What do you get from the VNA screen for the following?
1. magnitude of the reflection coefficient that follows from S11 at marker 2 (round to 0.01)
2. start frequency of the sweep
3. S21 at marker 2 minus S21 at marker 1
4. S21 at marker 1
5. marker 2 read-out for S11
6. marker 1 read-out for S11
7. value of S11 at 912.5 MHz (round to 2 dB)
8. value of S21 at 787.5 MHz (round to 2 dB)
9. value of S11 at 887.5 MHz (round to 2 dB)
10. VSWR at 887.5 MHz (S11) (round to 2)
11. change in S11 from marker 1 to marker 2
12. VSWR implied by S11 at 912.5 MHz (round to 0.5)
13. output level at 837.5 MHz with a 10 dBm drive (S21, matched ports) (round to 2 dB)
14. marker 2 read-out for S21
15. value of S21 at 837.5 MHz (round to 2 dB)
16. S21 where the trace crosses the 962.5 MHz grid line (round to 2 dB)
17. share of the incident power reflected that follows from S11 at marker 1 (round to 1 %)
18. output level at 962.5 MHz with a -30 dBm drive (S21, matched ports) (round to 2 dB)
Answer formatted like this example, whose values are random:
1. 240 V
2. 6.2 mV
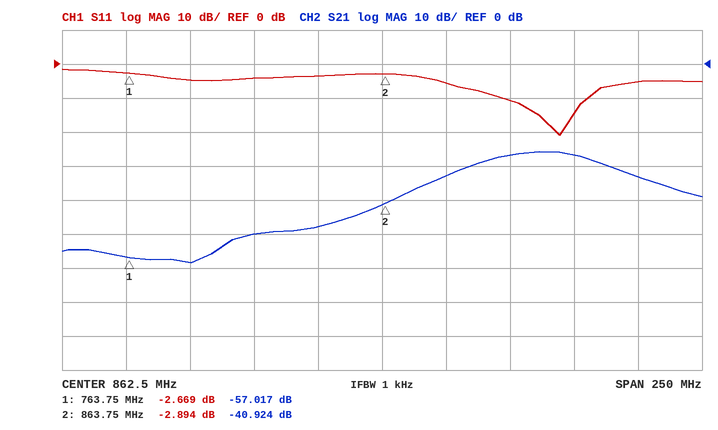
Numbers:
1. 0.72
2. 737.5 MHz
3. 16.093 dB
4. -57.017 dB
5. -2.894 dB
6. -2.669 dB
7. -10 dB
8. -58 dB
9. -6 dB
10. 4
11. -0.225 dB
12. 2.0
13. -38 dBm
14. -40.924 dB
15. -48 dB
16. -34 dB
17. 54 %
18. -64 dBm
